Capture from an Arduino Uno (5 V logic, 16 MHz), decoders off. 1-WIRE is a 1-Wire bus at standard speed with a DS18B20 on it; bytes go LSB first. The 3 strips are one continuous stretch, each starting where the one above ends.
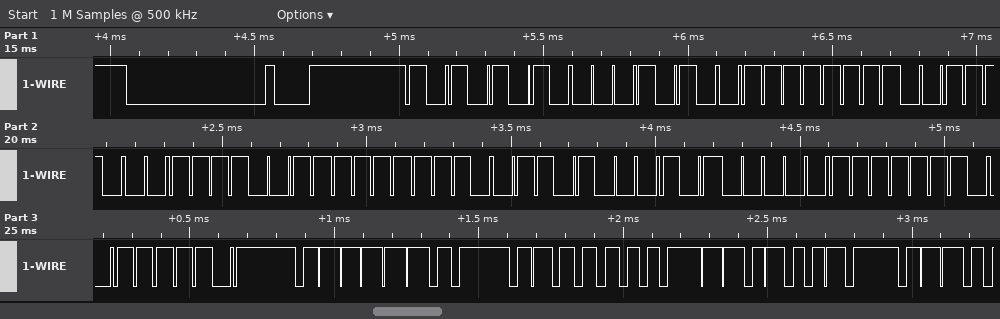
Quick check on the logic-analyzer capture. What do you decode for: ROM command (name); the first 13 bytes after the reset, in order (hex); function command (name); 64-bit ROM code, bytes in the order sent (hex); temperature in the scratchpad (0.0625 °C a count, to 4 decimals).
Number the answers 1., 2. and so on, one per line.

1. Match ROM
2. 55 28 FF 1C CF 7F 16 05 7F BE 3E 02 4B
3. Read Scratchpad
4. 28 FF 1C CF 7F 16 05 7F
5. 35.8750 °C
